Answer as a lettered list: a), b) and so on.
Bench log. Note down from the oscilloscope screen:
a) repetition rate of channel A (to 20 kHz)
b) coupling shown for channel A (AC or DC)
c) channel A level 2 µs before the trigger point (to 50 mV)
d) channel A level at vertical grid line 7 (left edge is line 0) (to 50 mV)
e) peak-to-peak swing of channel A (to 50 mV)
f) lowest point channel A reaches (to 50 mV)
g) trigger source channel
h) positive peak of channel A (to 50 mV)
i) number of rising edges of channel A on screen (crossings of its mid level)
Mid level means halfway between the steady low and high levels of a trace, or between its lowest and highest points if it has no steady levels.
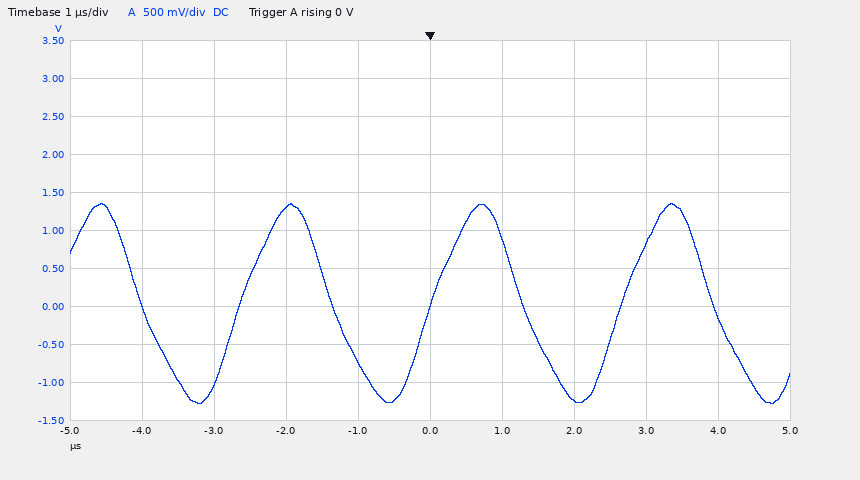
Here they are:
a) 380 kHz
b) DC
c) 1.30 V
d) -1.25 V
e) 2.65 V
f) -1.30 V
g) channel A
h) 1.35 V
i) 3
